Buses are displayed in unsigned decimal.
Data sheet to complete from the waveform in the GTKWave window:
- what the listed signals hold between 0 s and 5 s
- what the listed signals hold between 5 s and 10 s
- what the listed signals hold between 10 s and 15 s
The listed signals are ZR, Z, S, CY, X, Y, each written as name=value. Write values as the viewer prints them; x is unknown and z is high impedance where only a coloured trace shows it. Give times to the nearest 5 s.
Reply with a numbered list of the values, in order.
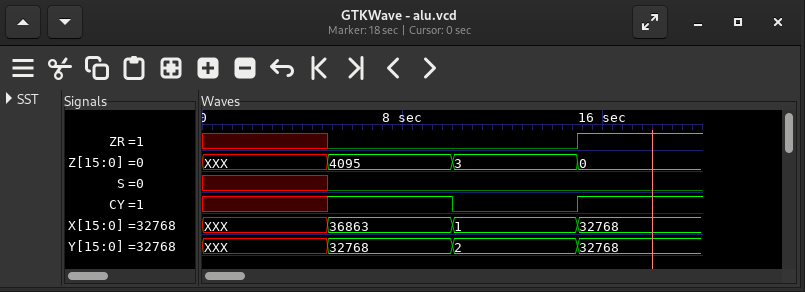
1. ZR=x, Z=XXX, S=x, CY=x, X=XXX, Y=XXX
2. ZR=0, Z=4095, S=0, CY=1, X=36863, Y=32768
3. ZR=0, Z=3, S=0, CY=0, X=1, Y=2
